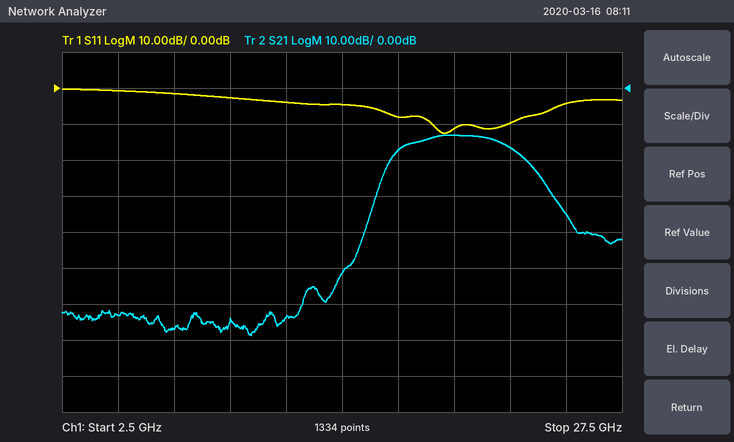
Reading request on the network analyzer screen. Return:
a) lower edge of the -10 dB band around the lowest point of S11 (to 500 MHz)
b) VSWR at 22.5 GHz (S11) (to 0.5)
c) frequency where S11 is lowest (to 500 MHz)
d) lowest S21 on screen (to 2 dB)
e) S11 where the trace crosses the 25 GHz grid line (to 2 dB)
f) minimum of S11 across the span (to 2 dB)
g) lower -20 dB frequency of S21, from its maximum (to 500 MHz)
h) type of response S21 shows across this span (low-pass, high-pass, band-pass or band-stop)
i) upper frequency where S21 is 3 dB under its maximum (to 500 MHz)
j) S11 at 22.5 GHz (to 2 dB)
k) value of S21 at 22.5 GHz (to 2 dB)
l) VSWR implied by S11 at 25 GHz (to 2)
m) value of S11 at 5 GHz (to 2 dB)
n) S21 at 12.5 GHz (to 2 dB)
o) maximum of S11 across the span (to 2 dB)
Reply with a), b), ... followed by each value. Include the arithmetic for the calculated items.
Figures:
a) 19.0 GHz
b) |Γ| = 10^(-10/20) = 0.3162; VSWR = (1 + 0.3162)/(1 − 0.3162) ≈ 1.92, so 2.0 to the nearest 0.5
c) 19.5 GHz
d) -68 dB
e) -4 dB
f) -12 dB
g) 16.5 GHz
h) band-pass
i) 22.5 GHz
j) -10 dB
k) -16 dB
l) |Γ| = 10^(-4/20) = 0.6310; VSWR = (1 + 0.6310)/(1 − 0.6310) ≈ 4
m) 0 dB
n) -64 dB
o) 0 dB
